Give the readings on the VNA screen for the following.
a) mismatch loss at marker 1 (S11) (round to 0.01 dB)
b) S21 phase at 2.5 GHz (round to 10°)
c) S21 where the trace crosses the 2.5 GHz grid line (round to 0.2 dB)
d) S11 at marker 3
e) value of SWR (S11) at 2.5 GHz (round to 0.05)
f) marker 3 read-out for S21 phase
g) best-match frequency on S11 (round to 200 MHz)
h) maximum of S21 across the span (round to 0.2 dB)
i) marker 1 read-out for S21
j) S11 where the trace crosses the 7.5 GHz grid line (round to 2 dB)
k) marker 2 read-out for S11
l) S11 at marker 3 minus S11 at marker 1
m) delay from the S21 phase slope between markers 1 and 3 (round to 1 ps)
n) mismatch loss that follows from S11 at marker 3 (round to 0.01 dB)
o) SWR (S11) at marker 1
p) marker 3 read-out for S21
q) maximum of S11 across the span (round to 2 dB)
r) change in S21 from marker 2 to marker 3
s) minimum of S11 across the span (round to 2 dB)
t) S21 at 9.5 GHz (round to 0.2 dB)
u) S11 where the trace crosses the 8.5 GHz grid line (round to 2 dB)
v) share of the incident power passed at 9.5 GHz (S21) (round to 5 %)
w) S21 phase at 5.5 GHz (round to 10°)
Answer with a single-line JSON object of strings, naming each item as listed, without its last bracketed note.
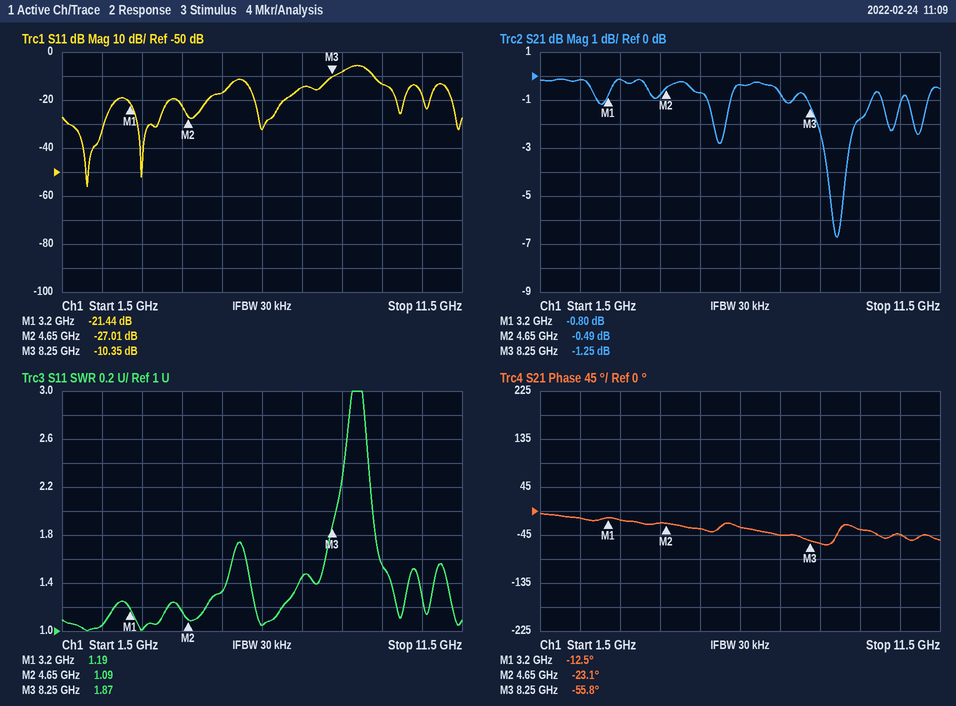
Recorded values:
{"mismatch loss at marker 1 (S11)": "0.03 dB", "S21 phase at 2.5 GHz": "-10°", "S21 where the trace crosses the 2.5 GHz grid line": "-0.2 dB", "S11 at marker 3": "-10.35 dB", "value of SWR (S11) at 2.5 GHz": "1.05", "marker 3 read-out for S21 phase": "-55.8°", "best-match frequency on S11": "2.2 GHz", "maximum of S21 across the span": "-0.2 dB", "marker 1 read-out for S21": "-0.80 dB", "S11 where the trace crosses the 7.5 GHz grid line": "-14 dB", "marker 2 read-out for S11": "-27.01 dB", "S11 at marker 3 minus S11 at marker 1": "11.09 dB", "delay from the S21 phase slope between markers 1 and 3": "24 ps", "mismatch loss that follows from S11 at marker 3": "0.42 dB", "SWR (S11) at marker 1": "1.19", "marker 3 read-out for S21": "-1.25 dB", "maximum of S11 across the span": "-6 dB", "change in S21 from marker 2 to marker 3": "-0.76 dB", "minimum of S11 across the span": "-56 dB", "S21 at 9.5 GHz": "-1.8 dB", "S11 where the trace crosses the 8.5 GHz grid line": "-8 dB", "share of the incident power passed at 9.5 GHz (S21)": "65 %", "S21 phase at 5.5 GHz": "-30°"}
